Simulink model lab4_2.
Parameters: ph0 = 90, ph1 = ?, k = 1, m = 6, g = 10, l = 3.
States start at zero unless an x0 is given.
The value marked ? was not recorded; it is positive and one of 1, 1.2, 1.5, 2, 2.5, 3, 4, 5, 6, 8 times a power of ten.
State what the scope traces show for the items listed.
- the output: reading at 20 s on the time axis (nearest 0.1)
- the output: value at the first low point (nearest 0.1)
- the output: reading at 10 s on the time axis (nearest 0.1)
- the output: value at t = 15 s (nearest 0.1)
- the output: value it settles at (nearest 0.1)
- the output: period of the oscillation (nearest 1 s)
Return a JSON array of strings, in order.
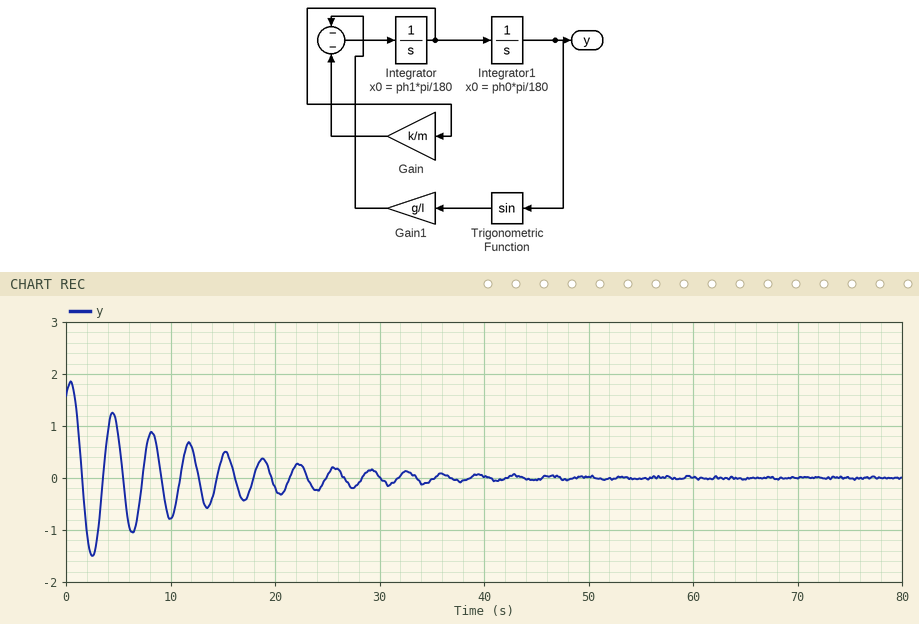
["-0.2", "-1.5", "-0.8", "0.4", "0.0", "4 s"]
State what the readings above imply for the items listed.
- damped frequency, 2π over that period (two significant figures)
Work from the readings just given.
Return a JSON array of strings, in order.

["1.6 rad/s"]
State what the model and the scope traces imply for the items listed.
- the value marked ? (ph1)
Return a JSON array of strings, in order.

["80"]
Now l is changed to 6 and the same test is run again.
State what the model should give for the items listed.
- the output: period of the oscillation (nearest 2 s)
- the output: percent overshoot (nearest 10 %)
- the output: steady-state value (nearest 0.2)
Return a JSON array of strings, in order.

["6 s", "100 %", "0.0"]
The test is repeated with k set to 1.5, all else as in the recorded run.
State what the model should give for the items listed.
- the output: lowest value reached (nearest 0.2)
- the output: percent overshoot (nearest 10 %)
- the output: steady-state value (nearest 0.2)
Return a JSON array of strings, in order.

["-1.4", "90 %", "0.0"]
